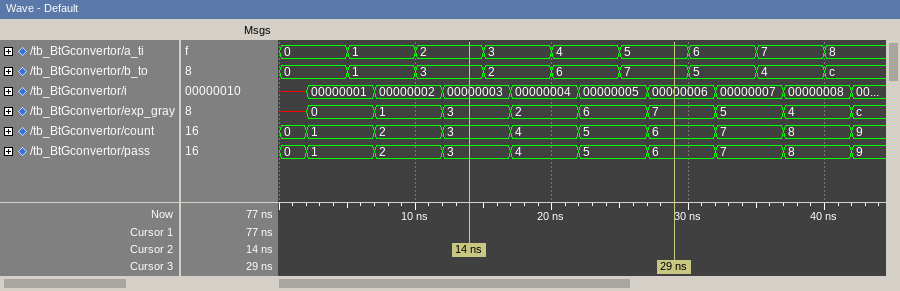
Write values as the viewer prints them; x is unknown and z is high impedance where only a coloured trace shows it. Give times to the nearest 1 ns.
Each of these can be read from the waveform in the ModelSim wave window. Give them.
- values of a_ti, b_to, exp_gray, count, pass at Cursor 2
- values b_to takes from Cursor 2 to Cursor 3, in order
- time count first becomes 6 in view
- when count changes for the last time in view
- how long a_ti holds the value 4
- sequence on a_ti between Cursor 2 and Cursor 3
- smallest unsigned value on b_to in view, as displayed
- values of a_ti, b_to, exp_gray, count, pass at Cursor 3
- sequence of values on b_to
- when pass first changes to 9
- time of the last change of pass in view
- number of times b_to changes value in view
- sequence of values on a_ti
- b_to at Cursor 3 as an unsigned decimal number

a_ti=2, b_to=3, exp_gray=3, count=3, pass=3
3, 2, 6, 7
27 ns
42 ns
5 ns
2, 3, 4, 5
0
a_ti=5, b_to=7, exp_gray=7, count=6, pass=6
0, 1, 3, 2, 6, 7, 5, 4, c
42 ns
42 ns
8
0, 1, 2, 3, 4, 5, 6, 7, 8
7
